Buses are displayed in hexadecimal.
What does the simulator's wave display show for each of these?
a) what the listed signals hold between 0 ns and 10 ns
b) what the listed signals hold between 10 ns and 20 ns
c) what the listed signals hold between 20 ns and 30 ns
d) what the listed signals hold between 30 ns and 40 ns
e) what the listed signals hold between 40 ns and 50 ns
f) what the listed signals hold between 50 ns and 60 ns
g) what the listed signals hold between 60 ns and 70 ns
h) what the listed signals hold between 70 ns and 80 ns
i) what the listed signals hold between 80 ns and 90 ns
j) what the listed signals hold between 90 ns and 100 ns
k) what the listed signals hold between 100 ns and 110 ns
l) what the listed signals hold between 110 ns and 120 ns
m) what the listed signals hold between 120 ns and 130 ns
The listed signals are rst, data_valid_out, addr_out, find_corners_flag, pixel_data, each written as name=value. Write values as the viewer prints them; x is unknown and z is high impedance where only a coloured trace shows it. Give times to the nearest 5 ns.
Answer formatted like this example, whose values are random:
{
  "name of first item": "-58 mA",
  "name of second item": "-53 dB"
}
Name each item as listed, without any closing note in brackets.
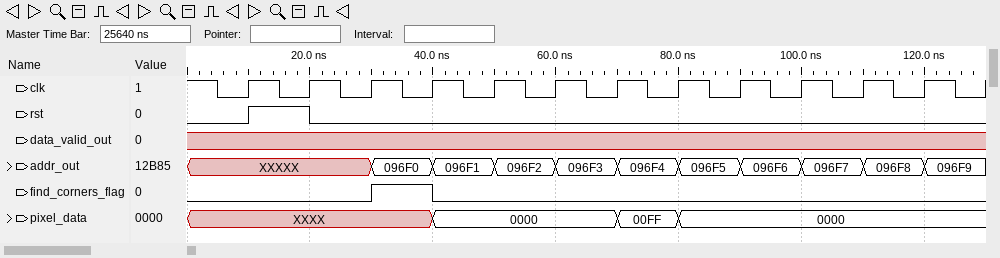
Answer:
{
  "what the listed signals hold between 0 ns and 10 ns": "rst=0, data_valid_out=x, addr_out=XXXXX, find_corners_flag=0, pixel_data=XXXX",
  "what the listed signals hold between 10 ns and 20 ns": "rst=1, data_valid_out=x, addr_out=XXXXX, find_corners_flag=0, pixel_data=XXXX",
  "what the listed signals hold between 20 ns and 30 ns": "rst=0, data_valid_out=x, addr_out=XXXXX, find_corners_flag=0, pixel_data=XXXX",
  "what the listed signals hold between 30 ns and 40 ns": "rst=0, data_valid_out=x, addr_out=096F0, find_corners_flag=1, pixel_data=XXXX",
  "what the listed signals hold between 40 ns and 50 ns": "rst=0, data_valid_out=x, addr_out=096F1, find_corners_flag=0, pixel_data=0000",
  "what the listed signals hold between 50 ns and 60 ns": "rst=0, data_valid_out=x, addr_out=096F2, find_corners_flag=0, pixel_data=0000",
  "what the listed signals hold between 60 ns and 70 ns": "rst=0, data_valid_out=x, addr_out=096F3, find_corners_flag=0, pixel_data=0000",
  "what the listed signals hold between 70 ns and 80 ns": "rst=0, data_valid_out=x, addr_out=096F4, find_corners_flag=0, pixel_data=00FF",
  "what the listed signals hold between 80 ns and 90 ns": "rst=0, data_valid_out=x, addr_out=096F5, find_corners_flag=0, pixel_data=0000",
  "what the listed signals hold between 90 ns and 100 ns": "rst=0, data_valid_out=x, addr_out=096F6, find_corners_flag=0, pixel_data=0000",
  "what the listed signals hold between 100 ns and 110 ns": "rst=0, data_valid_out=x, addr_out=096F7, find_corners_flag=0, pixel_data=0000",
  "what the listed signals hold between 110 ns and 120 ns": "rst=0, data_valid_out=x, addr_out=096F8, find_corners_flag=0, pixel_data=0000",
  "what the listed signals hold between 120 ns and 130 ns": "rst=0, data_valid_out=x, addr_out=096F9, find_corners_flag=0, pixel_data=0000"
}
